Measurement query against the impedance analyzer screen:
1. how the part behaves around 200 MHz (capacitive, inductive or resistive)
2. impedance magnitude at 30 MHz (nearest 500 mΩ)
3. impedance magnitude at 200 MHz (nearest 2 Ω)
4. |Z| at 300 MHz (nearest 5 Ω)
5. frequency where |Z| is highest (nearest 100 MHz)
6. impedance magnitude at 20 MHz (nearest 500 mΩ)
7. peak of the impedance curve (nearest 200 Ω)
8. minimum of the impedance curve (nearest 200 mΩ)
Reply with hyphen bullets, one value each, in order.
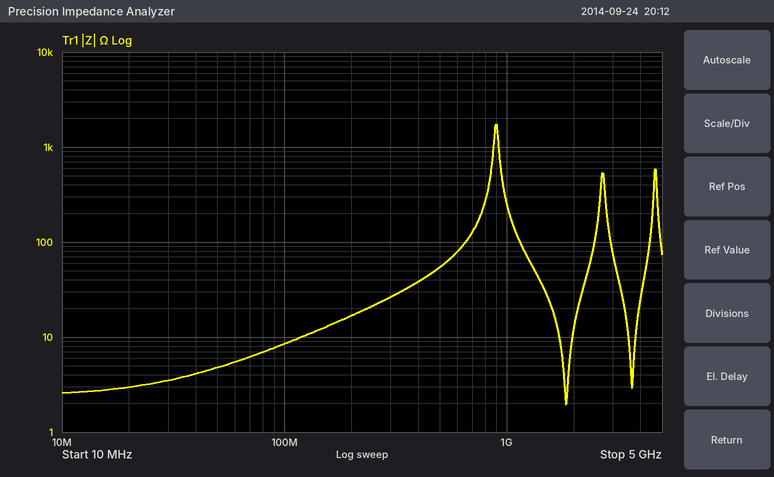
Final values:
- inductive
- 3.5 Ω
- 16 Ω
- 25 Ω
- 900 MHz
- 3.0 Ω
- 1.8 kΩ
- 2.0 Ω
